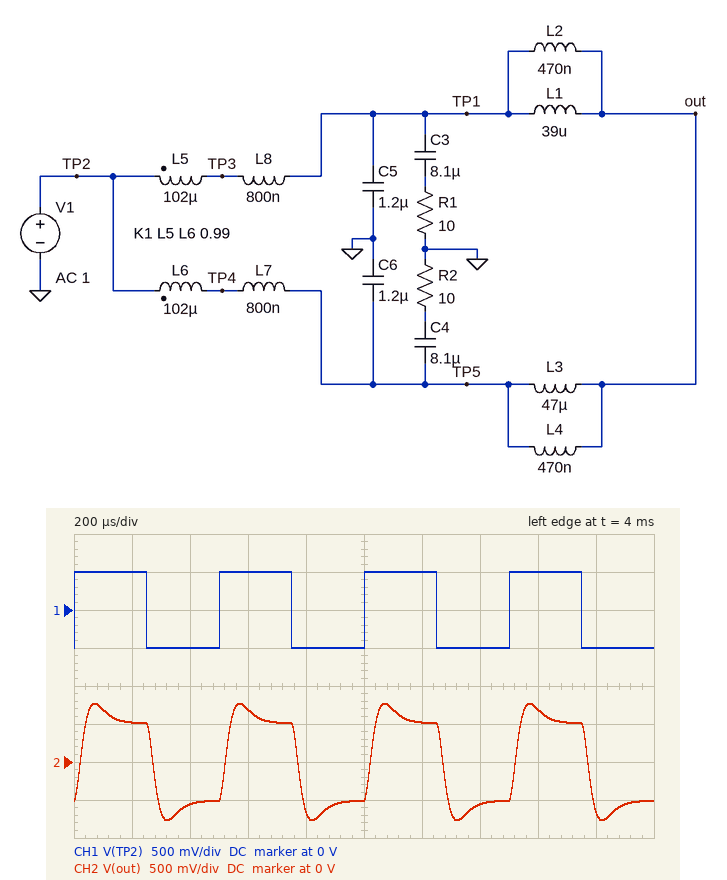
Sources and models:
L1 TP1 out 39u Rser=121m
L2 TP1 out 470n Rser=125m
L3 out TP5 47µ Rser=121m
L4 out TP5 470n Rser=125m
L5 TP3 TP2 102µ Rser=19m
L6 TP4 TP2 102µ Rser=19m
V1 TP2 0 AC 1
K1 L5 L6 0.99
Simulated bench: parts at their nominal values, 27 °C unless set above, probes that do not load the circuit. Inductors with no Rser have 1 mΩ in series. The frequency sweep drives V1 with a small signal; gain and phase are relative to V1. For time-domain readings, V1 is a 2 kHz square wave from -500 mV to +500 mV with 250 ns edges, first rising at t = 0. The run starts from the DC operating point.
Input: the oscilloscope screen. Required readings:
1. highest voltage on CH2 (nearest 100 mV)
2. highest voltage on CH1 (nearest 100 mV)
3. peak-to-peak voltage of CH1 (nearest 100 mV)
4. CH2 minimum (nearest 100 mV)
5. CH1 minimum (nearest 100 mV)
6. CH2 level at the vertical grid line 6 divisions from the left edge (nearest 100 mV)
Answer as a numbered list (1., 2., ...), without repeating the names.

1. 800 mV
2. 500 mV
3. 1.0 V
4. -800 mV
5. -500 mV
6. 500 mV
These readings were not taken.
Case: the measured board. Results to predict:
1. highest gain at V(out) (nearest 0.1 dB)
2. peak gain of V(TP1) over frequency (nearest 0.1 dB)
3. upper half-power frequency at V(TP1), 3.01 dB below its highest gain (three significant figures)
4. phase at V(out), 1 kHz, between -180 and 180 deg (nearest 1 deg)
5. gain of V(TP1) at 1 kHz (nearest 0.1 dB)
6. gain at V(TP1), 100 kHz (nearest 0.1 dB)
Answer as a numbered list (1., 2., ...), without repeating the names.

1. 2.3 dB
2. 2.3 dB
3. 8.86 kHz
4. -2 deg
5. 0.5 dB
6. -39.7 dB
